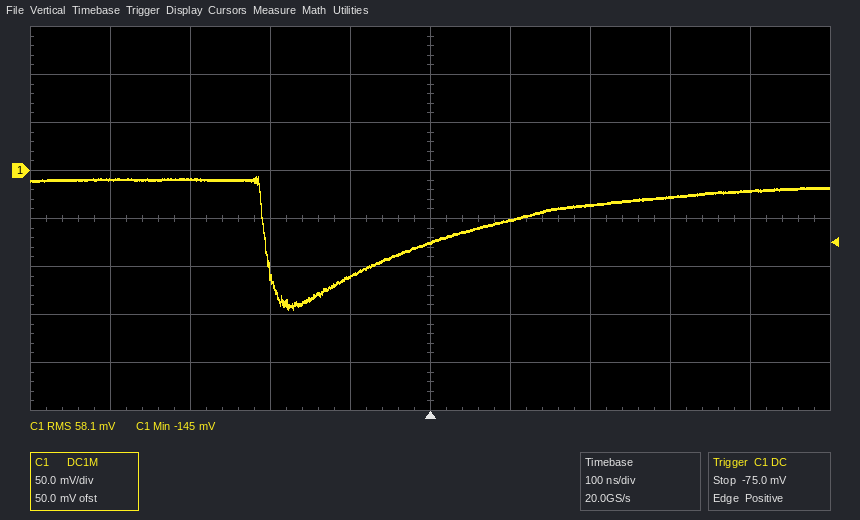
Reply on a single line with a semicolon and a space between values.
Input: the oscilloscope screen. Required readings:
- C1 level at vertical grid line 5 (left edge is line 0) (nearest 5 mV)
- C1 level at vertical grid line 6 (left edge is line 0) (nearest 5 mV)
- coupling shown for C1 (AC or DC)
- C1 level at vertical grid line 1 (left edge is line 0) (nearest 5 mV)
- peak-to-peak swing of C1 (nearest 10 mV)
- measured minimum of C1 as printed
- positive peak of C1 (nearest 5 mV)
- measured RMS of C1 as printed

-75 mV; -50 mV; DC; -10 mV; 140 mV; -145 mV; -5 mV; 58.1 mV
